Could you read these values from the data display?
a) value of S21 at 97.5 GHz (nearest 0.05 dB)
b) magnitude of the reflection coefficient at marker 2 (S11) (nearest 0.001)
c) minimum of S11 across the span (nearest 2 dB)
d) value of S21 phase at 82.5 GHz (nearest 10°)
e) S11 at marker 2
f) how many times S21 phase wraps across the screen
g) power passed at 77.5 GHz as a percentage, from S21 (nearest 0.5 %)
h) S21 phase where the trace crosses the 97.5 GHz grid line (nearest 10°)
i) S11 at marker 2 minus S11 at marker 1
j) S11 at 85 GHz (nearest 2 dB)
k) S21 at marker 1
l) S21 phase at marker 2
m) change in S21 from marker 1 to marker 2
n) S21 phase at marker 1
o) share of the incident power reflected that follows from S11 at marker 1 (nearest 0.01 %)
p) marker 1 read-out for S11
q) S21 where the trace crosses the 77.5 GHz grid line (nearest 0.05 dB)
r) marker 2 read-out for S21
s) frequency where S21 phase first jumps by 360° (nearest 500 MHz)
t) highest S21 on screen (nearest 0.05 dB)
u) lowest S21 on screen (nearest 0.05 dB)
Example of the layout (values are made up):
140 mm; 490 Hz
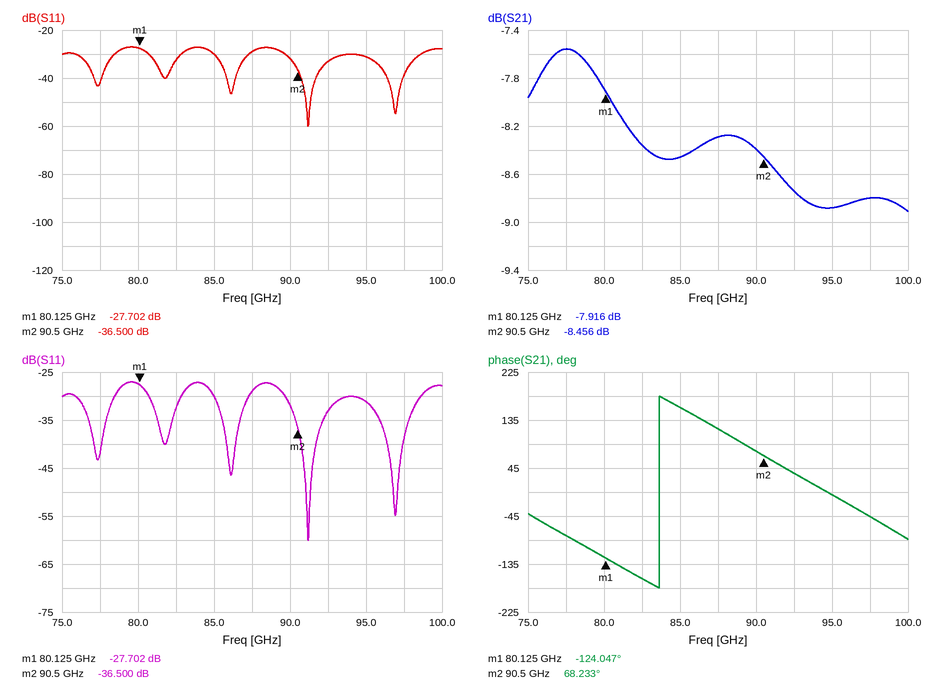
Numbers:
-8.80 dB; 0.015; -60 dB; -160°; -36.500 dB; 1; 17.5 %; -50°; -8.798 dB; -30 dB; -7.916 dB; 68.233°; -0.540 dB; -124.047°; 0.17 %; -27.702 dB; -7.55 dB; -8.456 dB; 83.5 GHz; -7.55 dB; -8.90 dB
